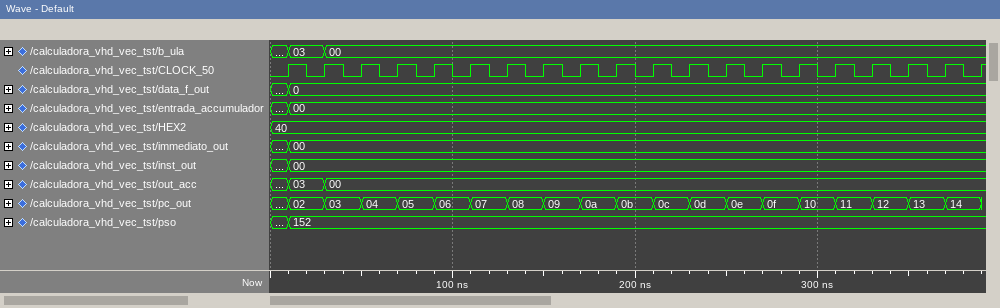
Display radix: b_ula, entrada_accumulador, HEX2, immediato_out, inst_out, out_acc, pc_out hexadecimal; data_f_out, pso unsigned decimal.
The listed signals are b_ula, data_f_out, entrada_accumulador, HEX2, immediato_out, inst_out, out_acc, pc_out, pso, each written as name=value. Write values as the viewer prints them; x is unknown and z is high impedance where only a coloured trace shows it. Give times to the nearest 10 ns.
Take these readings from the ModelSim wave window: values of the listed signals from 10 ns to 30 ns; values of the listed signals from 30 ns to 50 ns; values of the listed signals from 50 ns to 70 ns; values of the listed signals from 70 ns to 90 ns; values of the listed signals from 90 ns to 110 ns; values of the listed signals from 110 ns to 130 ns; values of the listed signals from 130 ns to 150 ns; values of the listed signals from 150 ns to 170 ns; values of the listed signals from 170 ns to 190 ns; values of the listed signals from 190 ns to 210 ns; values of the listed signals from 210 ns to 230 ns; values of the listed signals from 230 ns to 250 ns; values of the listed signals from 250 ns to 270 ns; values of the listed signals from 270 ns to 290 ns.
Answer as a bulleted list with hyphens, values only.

- b_ula=03, data_f_out=0, entrada_accumulador=00, HEX2=40, immediato_out=00, inst_out=00, out_acc=03, pc_out=02, pso=152
- b_ula=00, data_f_out=0, entrada_accumulador=00, HEX2=40, immediato_out=00, inst_out=00, out_acc=00, pc_out=03, pso=152
- b_ula=00, data_f_out=0, entrada_accumulador=00, HEX2=40, immediato_out=00, inst_out=00, out_acc=00, pc_out=04, pso=152
- b_ula=00, data_f_out=0, entrada_accumulador=00, HEX2=40, immediato_out=00, inst_out=00, out_acc=00, pc_out=05, pso=152
- b_ula=00, data_f_out=0, entrada_accumulador=00, HEX2=40, immediato_out=00, inst_out=00, out_acc=00, pc_out=06, pso=152
- b_ula=00, data_f_out=0, entrada_accumulador=00, HEX2=40, immediato_out=00, inst_out=00, out_acc=00, pc_out=07, pso=152
- b_ula=00, data_f_out=0, entrada_accumulador=00, HEX2=40, immediato_out=00, inst_out=00, out_acc=00, pc_out=08, pso=152
- b_ula=00, data_f_out=0, entrada_accumulador=00, HEX2=40, immediato_out=00, inst_out=00, out_acc=00, pc_out=09, pso=152
- b_ula=00, data_f_out=0, entrada_accumulador=00, HEX2=40, immediato_out=00, inst_out=00, out_acc=00, pc_out=0a, pso=152
- b_ula=00, data_f_out=0, entrada_accumulador=00, HEX2=40, immediato_out=00, inst_out=00, out_acc=00, pc_out=0b, pso=152
- b_ula=00, data_f_out=0, entrada_accumulador=00, HEX2=40, immediato_out=00, inst_out=00, out_acc=00, pc_out=0c, pso=152
- b_ula=00, data_f_out=0, entrada_accumulador=00, HEX2=40, immediato_out=00, inst_out=00, out_acc=00, pc_out=0d, pso=152
- b_ula=00, data_f_out=0, entrada_accumulador=00, HEX2=40, immediato_out=00, inst_out=00, out_acc=00, pc_out=0e, pso=152
- b_ula=00, data_f_out=0, entrada_accumulador=00, HEX2=40, immediato_out=00, inst_out=00, out_acc=00, pc_out=0f, pso=152
